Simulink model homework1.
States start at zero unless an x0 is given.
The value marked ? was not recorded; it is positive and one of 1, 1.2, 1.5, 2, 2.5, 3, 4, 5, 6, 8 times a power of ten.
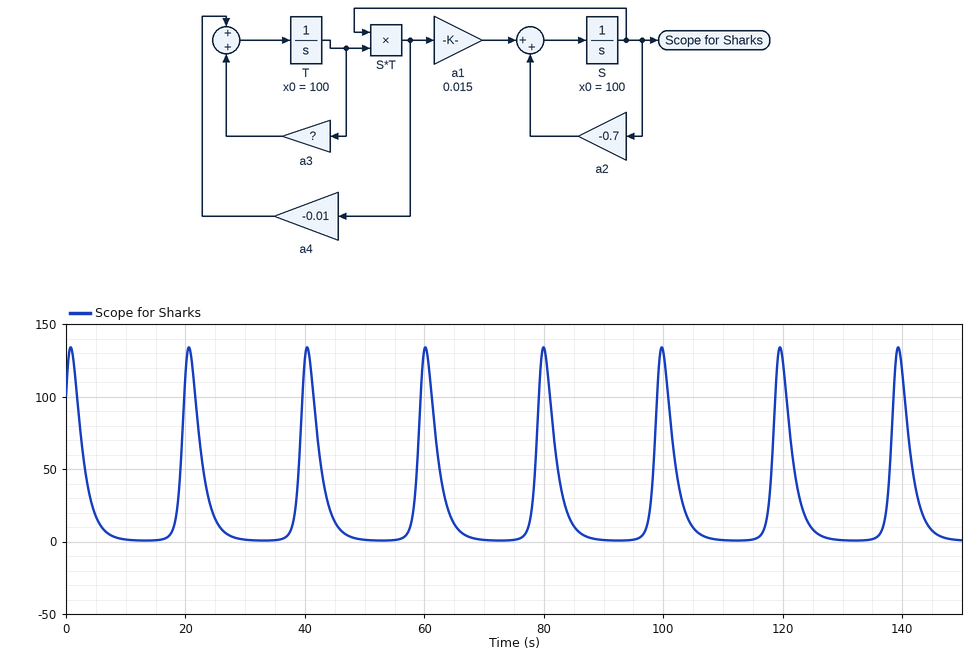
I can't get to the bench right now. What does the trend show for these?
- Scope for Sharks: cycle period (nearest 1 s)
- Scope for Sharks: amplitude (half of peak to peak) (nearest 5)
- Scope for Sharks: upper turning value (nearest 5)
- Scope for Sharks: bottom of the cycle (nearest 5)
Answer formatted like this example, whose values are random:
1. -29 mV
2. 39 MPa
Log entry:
1. 20 s
2. 65
3. 135
4. 0
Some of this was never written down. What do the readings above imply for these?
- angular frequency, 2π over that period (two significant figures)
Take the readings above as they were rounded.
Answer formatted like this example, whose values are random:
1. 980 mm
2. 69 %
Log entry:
1. 0.31 rad/s
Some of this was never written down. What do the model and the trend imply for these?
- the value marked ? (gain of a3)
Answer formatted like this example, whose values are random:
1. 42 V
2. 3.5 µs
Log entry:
1. 0.25
